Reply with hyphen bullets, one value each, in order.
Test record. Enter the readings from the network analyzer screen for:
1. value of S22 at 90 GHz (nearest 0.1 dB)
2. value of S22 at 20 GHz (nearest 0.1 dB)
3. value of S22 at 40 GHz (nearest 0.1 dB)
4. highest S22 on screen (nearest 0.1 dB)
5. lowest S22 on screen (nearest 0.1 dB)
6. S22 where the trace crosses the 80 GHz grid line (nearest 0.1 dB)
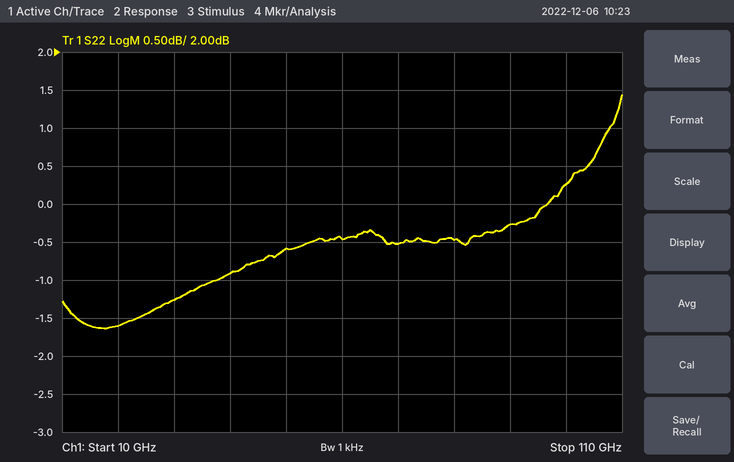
- -0.3 dB
- -1.6 dB
- -0.9 dB
- 1.4 dB
- -1.6 dB
- -0.5 dB
